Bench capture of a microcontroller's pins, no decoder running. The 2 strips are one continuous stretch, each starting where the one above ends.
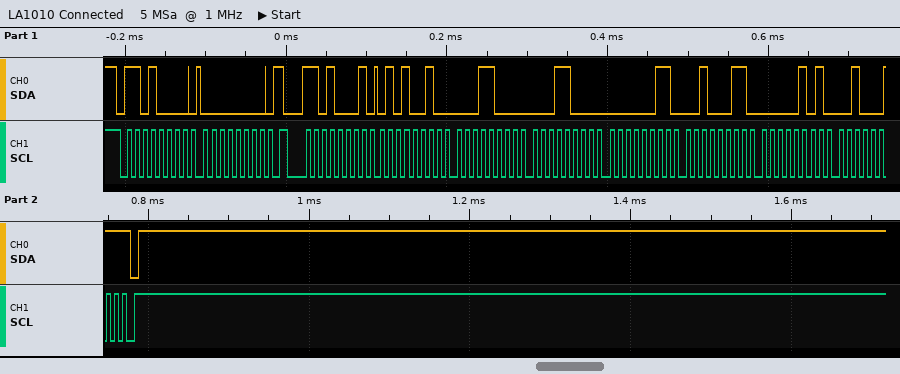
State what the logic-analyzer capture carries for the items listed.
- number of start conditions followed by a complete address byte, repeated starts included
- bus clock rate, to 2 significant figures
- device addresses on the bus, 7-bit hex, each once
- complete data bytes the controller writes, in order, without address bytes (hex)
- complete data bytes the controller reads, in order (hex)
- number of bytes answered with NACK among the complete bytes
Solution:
2
100 kHz
0x68
00
52 18 18 03 23 05 23
1
